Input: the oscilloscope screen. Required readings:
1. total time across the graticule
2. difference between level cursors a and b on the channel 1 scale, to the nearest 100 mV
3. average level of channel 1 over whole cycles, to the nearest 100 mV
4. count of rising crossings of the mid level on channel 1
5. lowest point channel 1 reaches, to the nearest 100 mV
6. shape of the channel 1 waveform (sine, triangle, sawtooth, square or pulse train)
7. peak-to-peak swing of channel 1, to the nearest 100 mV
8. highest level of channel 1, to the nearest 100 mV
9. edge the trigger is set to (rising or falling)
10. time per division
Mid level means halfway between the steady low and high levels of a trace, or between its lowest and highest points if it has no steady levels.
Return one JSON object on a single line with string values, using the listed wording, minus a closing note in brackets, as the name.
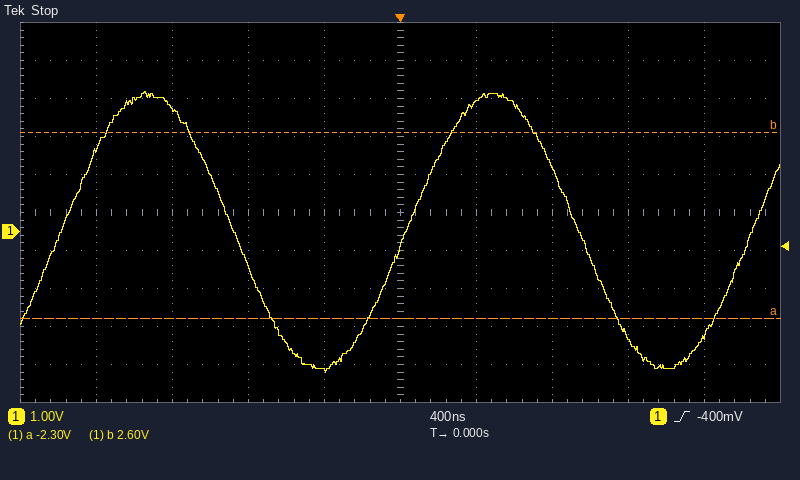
{"total time across the graticule": "4 µs", "difference between level cursors a and b on the channel 1 scale, to the nearest 100 mV": "4.9 V", "average level of channel 1 over whole cycles, to the nearest 100 mV": "0.0 V", "count of rising crossings of the mid level on channel 1": "3", "lowest point channel 1 reaches, to the nearest 100 mV": "-3.7 V", "shape of the channel 1 waveform": "sine", "peak-to-peak swing of channel 1, to the nearest 100 mV": "7.4 V", "highest level of channel 1, to the nearest 100 mV": "3.7 V", "edge the trigger is set to": "rising", "time per division": "400 ns"}
